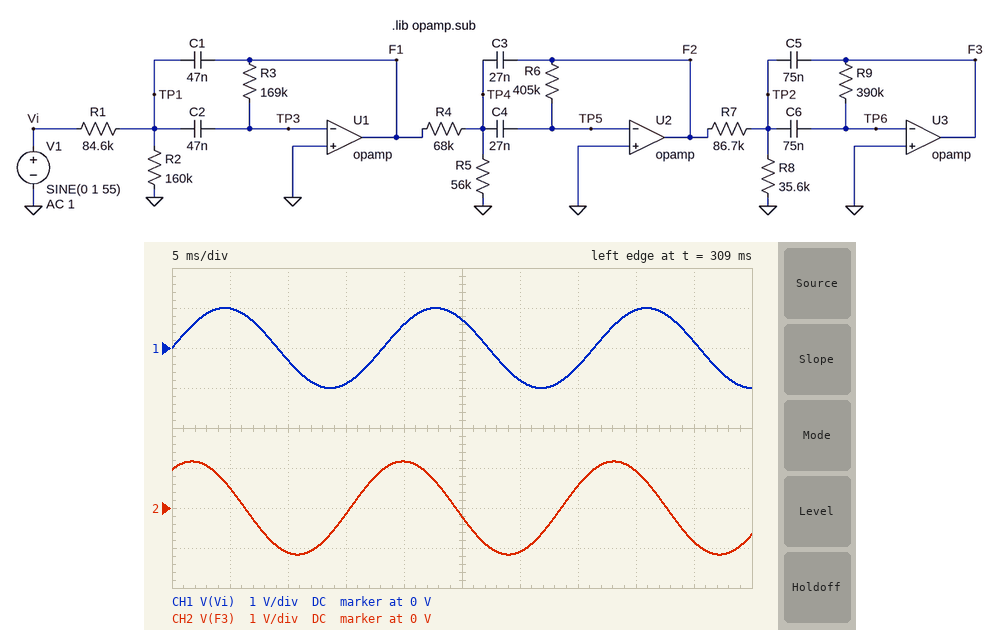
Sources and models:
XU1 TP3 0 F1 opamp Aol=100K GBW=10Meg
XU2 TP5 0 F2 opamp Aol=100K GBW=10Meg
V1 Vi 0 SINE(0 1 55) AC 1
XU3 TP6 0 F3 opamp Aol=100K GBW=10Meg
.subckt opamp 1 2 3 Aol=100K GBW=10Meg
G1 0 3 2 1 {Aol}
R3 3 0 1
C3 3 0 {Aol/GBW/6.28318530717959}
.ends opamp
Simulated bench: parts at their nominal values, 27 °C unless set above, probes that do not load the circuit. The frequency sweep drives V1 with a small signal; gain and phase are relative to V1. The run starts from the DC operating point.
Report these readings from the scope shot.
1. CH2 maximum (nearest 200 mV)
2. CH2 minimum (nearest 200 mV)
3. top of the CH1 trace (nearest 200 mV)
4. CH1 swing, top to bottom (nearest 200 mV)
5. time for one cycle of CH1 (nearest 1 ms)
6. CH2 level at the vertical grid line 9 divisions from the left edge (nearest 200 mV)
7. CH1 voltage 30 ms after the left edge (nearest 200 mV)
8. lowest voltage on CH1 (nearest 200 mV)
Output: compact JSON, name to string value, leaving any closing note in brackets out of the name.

{"CH2 maximum": "1.2 V", "CH2 minimum": "-1.2 V", "top of the CH1 trace": "1.0 V", "CH1 swing, top to bottom": "2.0 V", "time for one cycle of CH1": "18 ms", "CH2 level at the vertical grid line 9 divisions from the left edge": "-800 mV", "CH1 voltage 30 ms after the left edge": "-800 mV", "lowest voltage on CH1": "-1.0 V"}
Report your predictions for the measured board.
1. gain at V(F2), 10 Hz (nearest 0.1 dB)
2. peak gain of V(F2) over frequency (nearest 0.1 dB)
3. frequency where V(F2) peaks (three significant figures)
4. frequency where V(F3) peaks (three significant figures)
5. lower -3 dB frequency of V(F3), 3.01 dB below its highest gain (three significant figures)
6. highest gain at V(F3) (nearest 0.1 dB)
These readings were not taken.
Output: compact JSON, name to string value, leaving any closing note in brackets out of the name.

{"gain at V(F2), 10 Hz": "-19.4 dB", "peak gain of V(F2) over frequency": "7.8 dB", "frequency where V(F2) peaks": "49.5 Hz", "frequency where V(F3) peaks": "37.7 Hz", "lower -3 dB frequency of V(F3), 3.01 dB below its highest gain": "20.5 Hz", "highest gain at V(F3)": "4.2 dB"}
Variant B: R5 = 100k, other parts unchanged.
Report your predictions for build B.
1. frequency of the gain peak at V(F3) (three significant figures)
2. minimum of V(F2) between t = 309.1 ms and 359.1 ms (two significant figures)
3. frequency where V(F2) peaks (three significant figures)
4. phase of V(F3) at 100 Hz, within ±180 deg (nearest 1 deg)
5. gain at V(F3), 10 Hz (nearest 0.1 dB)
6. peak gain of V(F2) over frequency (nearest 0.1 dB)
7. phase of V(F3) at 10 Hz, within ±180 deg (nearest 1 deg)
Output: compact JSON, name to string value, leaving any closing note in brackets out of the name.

{"frequency of the gain peak at V(F3)": "32.9 Hz", "minimum of V(F2) between t = 309.1 ms and 359.1 ms": "-2.0 V", "frequency where V(F2) peaks": "43.3 Hz", "phase of V(F3) at 100 Hz, within ±180 deg": "-39 deg", "gain at V(F3), 10 Hz": "-20.6 dB", "peak gain of V(F2) over frequency": "8.7 dB", "phase of V(F3) at 10 Hz, within ±180 deg": "45 deg"}
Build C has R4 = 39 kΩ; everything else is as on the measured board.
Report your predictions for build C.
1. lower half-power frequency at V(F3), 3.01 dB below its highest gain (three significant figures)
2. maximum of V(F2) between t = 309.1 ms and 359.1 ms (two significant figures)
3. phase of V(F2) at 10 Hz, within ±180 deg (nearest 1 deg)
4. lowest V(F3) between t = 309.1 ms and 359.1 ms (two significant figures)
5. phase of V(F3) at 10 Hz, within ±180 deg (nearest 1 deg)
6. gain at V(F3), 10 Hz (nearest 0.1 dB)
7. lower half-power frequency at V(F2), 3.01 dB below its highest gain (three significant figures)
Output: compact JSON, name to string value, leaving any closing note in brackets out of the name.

{"lower half-power frequency at V(F3), 3.01 dB below its highest gain": "20.2 Hz", "maximum of V(F2) between t = 309.1 ms and 359.1 ms": "3.7 V", "phase of V(F2) at 10 Hz, within ±180 deg": "156 deg", "lowest V(F3) between t = 309.1 ms and 359.1 ms": "-1.9 V", "phase of V(F3) at 10 Hz, within ±180 deg": "49 deg", "gain at V(F3), 10 Hz": "-20.8 dB", "lower half-power frequency at V(F2), 3.01 dB below its highest gain": "42.3 Hz"}
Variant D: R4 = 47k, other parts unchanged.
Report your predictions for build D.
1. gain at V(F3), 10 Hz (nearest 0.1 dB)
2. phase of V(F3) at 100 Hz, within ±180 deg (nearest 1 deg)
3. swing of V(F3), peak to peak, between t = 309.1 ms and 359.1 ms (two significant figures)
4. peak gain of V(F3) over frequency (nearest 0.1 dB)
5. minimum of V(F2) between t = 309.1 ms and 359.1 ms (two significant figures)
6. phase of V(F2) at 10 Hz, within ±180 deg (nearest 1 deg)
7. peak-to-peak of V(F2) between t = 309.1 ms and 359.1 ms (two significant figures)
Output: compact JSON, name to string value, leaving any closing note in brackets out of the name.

{"gain at V(F3), 10 Hz": "-21.5 dB", "phase of V(F3) at 100 Hz, within ±180 deg": "-35 deg", "swing of V(F3), peak to peak, between t = 309.1 ms and 359.1 ms": "3.3 V", "peak gain of V(F3) over frequency": "5.4 dB", "minimum of V(F2) between t = 309.1 ms and 359.1 ms": "-3.3 V", "phase of V(F2) at 10 Hz, within ±180 deg": "155 deg", "peak-to-peak of V(F2) between t = 309.1 ms and 359.1 ms": "6.5 V"}
